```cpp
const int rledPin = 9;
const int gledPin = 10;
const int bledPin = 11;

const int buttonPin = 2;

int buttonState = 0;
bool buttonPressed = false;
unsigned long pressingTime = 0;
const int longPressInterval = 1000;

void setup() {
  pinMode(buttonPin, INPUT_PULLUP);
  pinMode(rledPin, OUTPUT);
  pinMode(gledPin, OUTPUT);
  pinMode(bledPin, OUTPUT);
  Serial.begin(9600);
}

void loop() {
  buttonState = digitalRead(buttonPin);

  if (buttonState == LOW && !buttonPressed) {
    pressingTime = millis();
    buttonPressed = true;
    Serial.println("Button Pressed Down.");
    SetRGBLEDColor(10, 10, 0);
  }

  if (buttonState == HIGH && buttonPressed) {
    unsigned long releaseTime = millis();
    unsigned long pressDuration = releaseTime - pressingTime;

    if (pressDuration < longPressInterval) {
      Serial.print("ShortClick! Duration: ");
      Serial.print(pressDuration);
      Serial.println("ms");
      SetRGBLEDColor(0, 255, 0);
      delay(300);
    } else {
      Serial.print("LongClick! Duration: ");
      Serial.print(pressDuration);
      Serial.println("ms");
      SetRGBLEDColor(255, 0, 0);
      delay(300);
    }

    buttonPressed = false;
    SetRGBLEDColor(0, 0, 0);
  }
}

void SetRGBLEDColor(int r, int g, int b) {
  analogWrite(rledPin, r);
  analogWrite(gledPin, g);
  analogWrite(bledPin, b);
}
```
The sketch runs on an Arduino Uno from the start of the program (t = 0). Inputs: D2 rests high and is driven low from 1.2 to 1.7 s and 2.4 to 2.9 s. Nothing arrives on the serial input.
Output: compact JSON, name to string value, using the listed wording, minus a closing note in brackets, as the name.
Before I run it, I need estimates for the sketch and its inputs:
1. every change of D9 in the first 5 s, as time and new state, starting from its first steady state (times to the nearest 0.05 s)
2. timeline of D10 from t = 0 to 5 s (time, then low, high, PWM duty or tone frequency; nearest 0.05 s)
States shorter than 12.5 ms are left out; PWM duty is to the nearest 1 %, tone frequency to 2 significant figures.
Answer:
{"every change of D9 in the first 5 s, as time and new state, starting from its first steady state": "0 s low; 1.2 s PWM 4 %; 1.7 s low; 2.4 s PWM 4 %; 2.9 s low", "timeline of D10 from t = 0 to 5 s": "0 s low; 1.2 s PWM 4 %; 1.7 s high; 2 s low; 2.4 s PWM 4 %; 2.9 s high; 3.2 s low"}
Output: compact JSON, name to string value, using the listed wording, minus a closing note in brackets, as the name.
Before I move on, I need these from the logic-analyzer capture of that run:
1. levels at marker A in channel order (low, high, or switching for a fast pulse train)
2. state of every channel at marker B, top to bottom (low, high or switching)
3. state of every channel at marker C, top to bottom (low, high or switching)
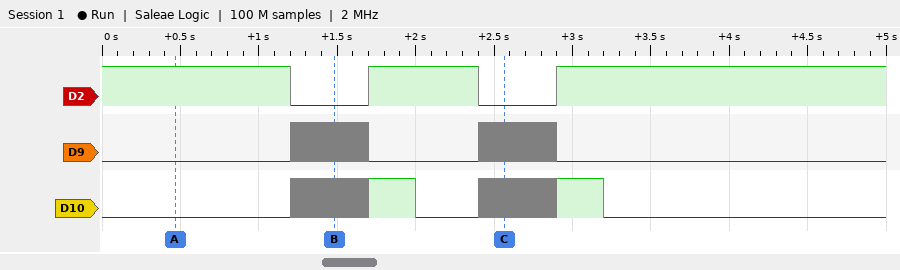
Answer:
{"levels at marker A in channel order": "D2 high, D9 low, D10 low", "state of every channel at marker B, top to bottom": "D2 low, D9 switching, D10 switching", "state of every channel at marker C, top to bottom": "D2 low, D9 switching, D10 switching"}
